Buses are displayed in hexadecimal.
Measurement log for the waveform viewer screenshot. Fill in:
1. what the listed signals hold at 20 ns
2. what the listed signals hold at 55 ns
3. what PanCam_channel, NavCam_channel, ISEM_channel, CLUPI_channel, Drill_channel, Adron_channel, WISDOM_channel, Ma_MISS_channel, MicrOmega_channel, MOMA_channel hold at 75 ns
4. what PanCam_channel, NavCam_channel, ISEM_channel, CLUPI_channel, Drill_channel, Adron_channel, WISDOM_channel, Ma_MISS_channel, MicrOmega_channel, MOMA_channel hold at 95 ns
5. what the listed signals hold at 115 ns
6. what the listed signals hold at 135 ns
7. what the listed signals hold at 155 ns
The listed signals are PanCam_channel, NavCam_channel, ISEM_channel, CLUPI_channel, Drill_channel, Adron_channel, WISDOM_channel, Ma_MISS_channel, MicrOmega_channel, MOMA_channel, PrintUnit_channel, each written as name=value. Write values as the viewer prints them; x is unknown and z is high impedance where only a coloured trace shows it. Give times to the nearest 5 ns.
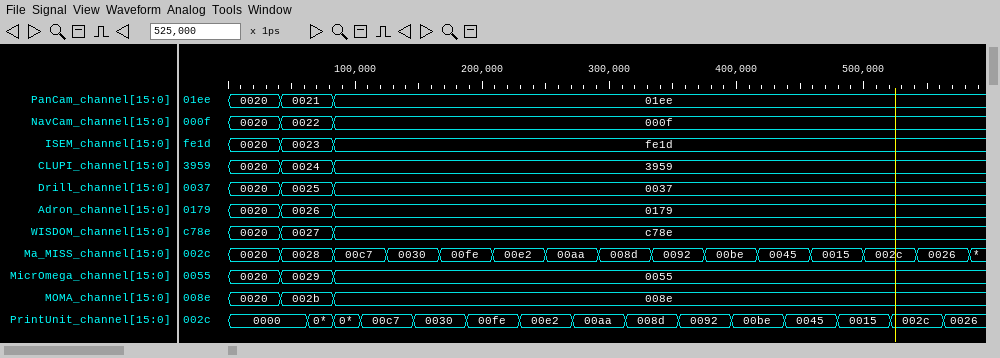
PanCam_channel=0020, NavCam_channel=0020, ISEM_channel=0020, CLUPI_channel=0020, Drill_channel=0020, Adron_channel=0020, WISDOM_channel=0020, Ma_MISS_channel=0020, MicrOmega_channel=0020, MOMA_channel=0020, PrintUnit_channel=0000
PanCam_channel=0021, NavCam_channel=0022, ISEM_channel=0023, CLUPI_channel=0024, Drill_channel=0025, Adron_channel=0026, WISDOM_channel=0027, Ma_MISS_channel=0028, MicrOmega_channel=0029, MOMA_channel=002b, PrintUnit_channel=0000
PanCam_channel=0021, NavCam_channel=0022, ISEM_channel=0023, CLUPI_channel=0024, Drill_channel=0025, Adron_channel=0026, WISDOM_channel=0027, Ma_MISS_channel=0028, MicrOmega_channel=0029, MOMA_channel=002b
PanCam_channel=01ee, NavCam_channel=000f, ISEM_channel=fe1d, CLUPI_channel=3959, Drill_channel=0037, Adron_channel=0179, WISDOM_channel=c78e, Ma_MISS_channel=00c7, MicrOmega_channel=0055, MOMA_channel=008e
PanCam_channel=01ee, NavCam_channel=000f, ISEM_channel=fe1d, CLUPI_channel=3959, Drill_channel=0037, Adron_channel=0179, WISDOM_channel=c78e, Ma_MISS_channel=00c7, MicrOmega_channel=0055, MOMA_channel=008e, PrintUnit_channel=00c7
PanCam_channel=01ee, NavCam_channel=000f, ISEM_channel=fe1d, CLUPI_channel=3959, Drill_channel=0037, Adron_channel=0179, WISDOM_channel=c78e, Ma_MISS_channel=0030, MicrOmega_channel=0055, MOMA_channel=008e, PrintUnit_channel=00c7
PanCam_channel=01ee, NavCam_channel=000f, ISEM_channel=fe1d, CLUPI_channel=3959, Drill_channel=0037, Adron_channel=0179, WISDOM_channel=c78e, Ma_MISS_channel=0030, MicrOmega_channel=0055, MOMA_channel=008e, PrintUnit_channel=0030
